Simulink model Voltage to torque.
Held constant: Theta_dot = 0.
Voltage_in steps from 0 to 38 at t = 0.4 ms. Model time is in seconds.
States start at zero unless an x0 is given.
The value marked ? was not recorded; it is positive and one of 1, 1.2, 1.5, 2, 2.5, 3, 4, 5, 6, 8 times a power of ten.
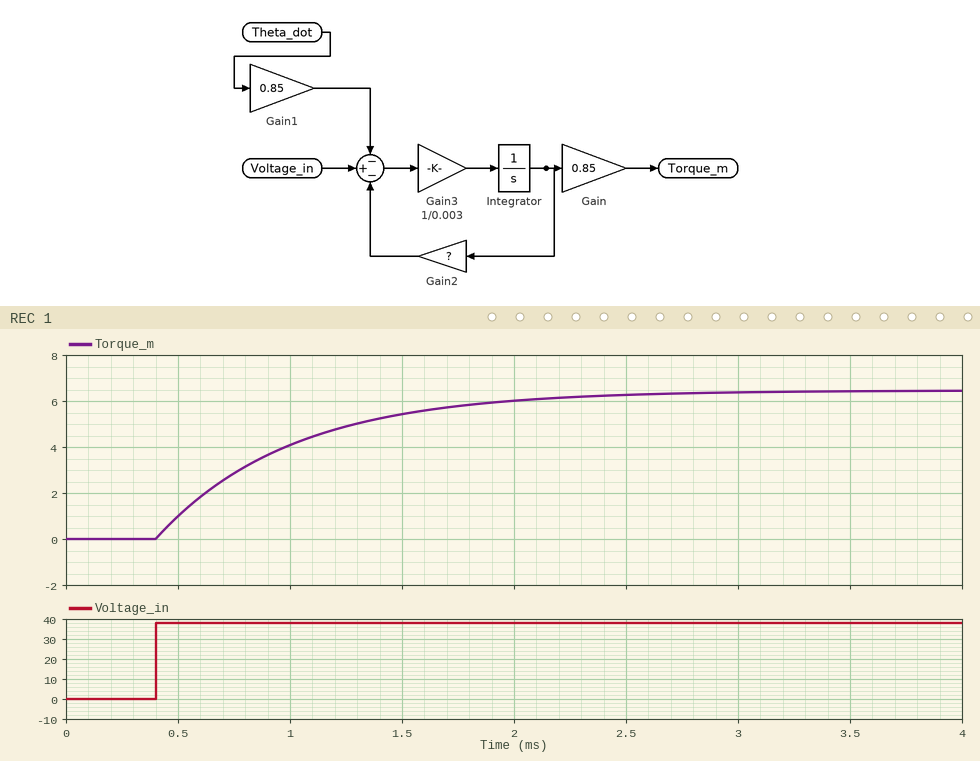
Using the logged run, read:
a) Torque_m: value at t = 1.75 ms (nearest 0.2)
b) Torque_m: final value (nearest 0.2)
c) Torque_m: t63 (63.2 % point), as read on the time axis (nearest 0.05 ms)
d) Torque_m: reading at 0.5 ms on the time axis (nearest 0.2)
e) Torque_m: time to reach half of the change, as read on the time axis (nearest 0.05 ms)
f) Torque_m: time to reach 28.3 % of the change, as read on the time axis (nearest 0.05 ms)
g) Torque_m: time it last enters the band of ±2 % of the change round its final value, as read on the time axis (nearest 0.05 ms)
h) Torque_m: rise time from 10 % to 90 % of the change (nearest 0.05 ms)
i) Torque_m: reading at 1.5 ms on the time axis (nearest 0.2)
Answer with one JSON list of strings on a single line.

["5.8", "6.4", "1.00 ms", "1.0", "0.80 ms", "0.60 ms", "2.75 ms", "1.30 ms", "5.4"]
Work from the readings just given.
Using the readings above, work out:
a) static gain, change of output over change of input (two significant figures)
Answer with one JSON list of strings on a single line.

["0.17"]
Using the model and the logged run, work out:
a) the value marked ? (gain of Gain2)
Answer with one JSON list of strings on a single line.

["5"]
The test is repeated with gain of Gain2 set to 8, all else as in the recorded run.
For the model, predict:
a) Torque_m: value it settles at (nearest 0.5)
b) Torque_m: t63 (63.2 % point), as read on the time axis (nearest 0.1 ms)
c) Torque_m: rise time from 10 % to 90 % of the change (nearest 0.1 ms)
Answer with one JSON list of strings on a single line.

["4.0", "0.8 ms", "0.8 ms"]
